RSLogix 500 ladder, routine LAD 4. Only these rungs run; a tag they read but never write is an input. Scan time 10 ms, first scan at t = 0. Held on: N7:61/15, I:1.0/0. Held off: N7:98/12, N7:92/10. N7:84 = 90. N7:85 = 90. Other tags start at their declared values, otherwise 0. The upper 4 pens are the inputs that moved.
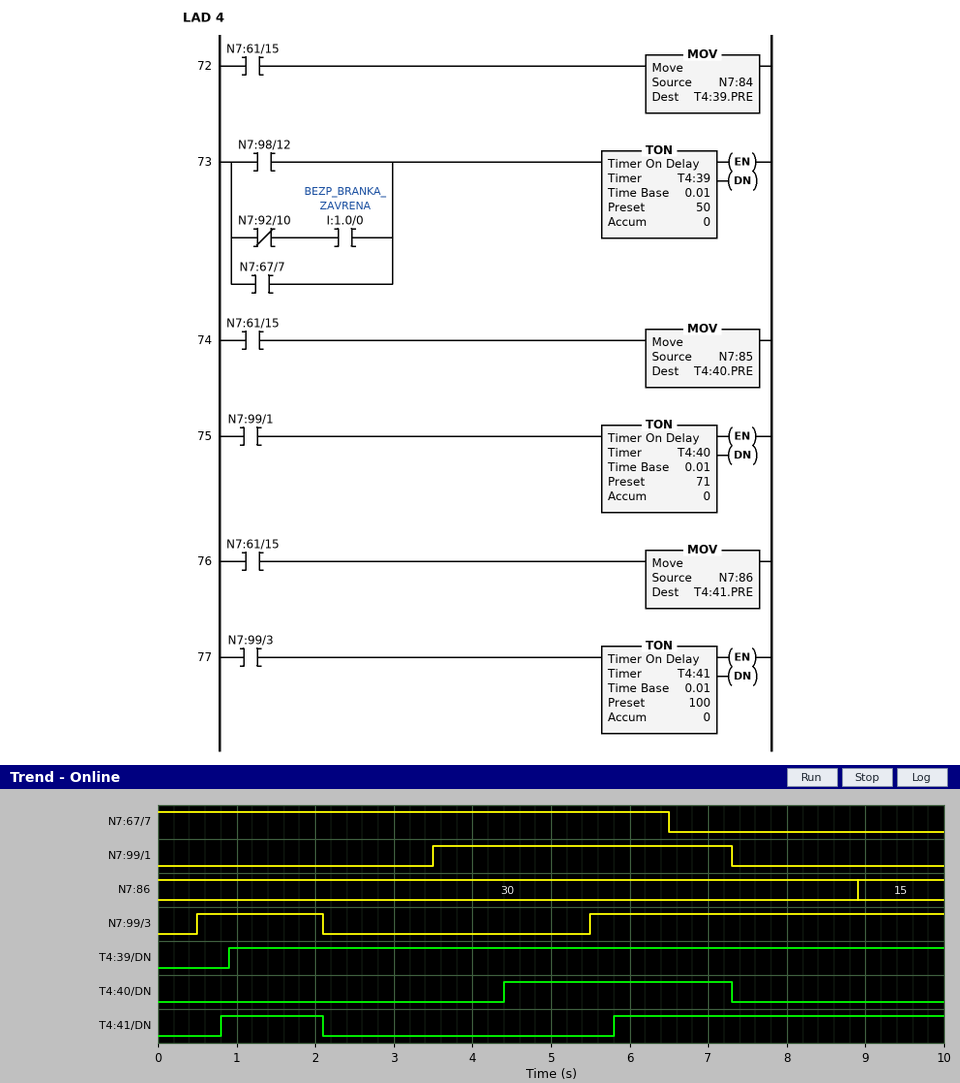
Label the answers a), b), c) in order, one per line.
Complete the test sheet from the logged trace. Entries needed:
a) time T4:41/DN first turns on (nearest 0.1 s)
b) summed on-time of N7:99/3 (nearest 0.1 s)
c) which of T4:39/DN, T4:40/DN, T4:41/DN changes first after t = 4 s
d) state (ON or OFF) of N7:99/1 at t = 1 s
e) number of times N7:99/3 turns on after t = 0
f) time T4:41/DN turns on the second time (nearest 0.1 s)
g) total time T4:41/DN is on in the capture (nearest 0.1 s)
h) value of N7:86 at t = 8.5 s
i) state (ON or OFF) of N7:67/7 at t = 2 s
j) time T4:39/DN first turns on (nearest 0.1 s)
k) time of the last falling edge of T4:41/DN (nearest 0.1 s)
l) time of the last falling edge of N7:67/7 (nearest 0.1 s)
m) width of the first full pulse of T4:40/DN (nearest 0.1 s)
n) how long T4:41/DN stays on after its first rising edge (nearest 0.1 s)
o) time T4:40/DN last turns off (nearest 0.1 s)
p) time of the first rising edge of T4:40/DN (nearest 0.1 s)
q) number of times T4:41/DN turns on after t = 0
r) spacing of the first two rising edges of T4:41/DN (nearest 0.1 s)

a) 0.8 s
b) 6.1 s
c) T4:40/DN
d) OFF
e) 2
f) 5.8 s
g) 5.5 s
h) 30
i) ON
j) 0.9 s
k) 2.1 s
l) 6.5 s
m) 2.9 s
n) 1.3 s
o) 7.3 s
p) 4.4 s
q) 2
r) 5.0 s
